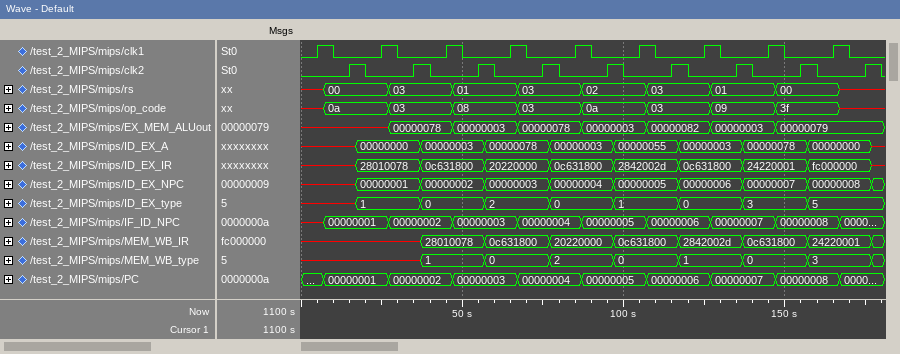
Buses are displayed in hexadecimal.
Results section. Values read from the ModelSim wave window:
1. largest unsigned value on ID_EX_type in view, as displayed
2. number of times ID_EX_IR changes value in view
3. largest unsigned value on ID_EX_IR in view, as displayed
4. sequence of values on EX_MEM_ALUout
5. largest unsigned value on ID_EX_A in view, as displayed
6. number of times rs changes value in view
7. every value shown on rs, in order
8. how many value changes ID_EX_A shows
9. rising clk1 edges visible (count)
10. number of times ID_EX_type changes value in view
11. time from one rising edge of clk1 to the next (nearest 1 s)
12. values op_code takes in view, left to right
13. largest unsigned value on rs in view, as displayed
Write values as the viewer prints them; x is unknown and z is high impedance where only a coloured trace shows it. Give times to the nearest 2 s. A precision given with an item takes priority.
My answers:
5
9
fc000000
x, 00000078, 00000003, 00000078, 00000003, 00000082, 00000003, 00000079
00000078
9
x, 00, 03, 01, 03, 02, 03, 01, 00, x
9
9
8
20 s
x, 0a, 03, 08, 03, 0a, 03, 09, 3f, x
03
